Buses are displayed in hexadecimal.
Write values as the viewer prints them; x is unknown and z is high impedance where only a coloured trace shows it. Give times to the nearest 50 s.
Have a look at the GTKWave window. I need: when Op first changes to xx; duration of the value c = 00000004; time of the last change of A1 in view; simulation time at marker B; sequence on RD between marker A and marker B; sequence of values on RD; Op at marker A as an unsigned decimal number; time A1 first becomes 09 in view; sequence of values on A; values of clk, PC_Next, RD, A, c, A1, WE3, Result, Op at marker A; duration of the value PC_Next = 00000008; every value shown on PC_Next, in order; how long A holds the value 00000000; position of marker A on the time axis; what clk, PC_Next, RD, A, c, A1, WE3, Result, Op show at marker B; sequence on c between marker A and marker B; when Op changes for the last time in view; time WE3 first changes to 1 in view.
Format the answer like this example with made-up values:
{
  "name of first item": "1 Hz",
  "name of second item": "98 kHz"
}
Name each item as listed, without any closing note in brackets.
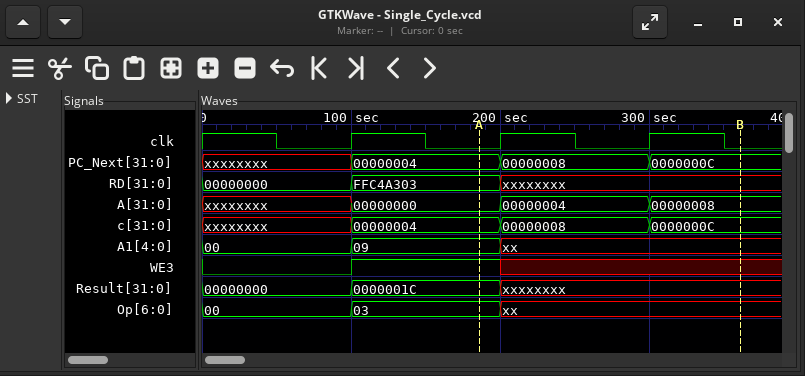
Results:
{
  "when Op first changes to xx": "200 s",
  "duration of the value c = 00000004": "100 s",
  "time of the last change of A1 in view": "200 s",
  "simulation time at marker B": "350 s",
  "sequence on RD between marker A and marker B": "FFC4A303, xxxxxxxx",
  "sequence of values on RD": "00000000, FFC4A303, xxxxxxxx",
  "Op at marker A as an unsigned decimal number": "3",
  "time A1 first becomes 09 in view": "100 s",
  "sequence of values on A": "xxxxxxxx, 00000000, 00000004, 00000008",
  "values of clk, PC_Next, RD, A, c, A1, WE3, Result, Op at marker A": "clk=0, PC_Next=00000004, RD=FFC4A303, A=00000000, c=00000004, A1=09, WE3=1, Result=0000001C, Op=03",
  "duration of the value PC_Next = 00000008": "100 s",
  "every value shown on PC_Next, in order": "xxxxxxxx, 00000004, 00000008, 0000000C",
  "how long A holds the value 00000000": "100 s",
  "position of marker A on the time axis": "200 s",
  "what clk, PC_Next, RD, A, c, A1, WE3, Result, Op show at marker B": "clk=0, PC_Next=0000000C, RD=xxxxxxxx, A=00000008, c=0000000C, A1=xx, WE3=x, Result=xxxxxxxx, Op=xx",
  "sequence on c between marker A and marker B": "00000004, 00000008, 0000000C",
  "when Op changes for the last time in view": "200 s",
  "time WE3 first changes to 1 in view": "100 s"
}
